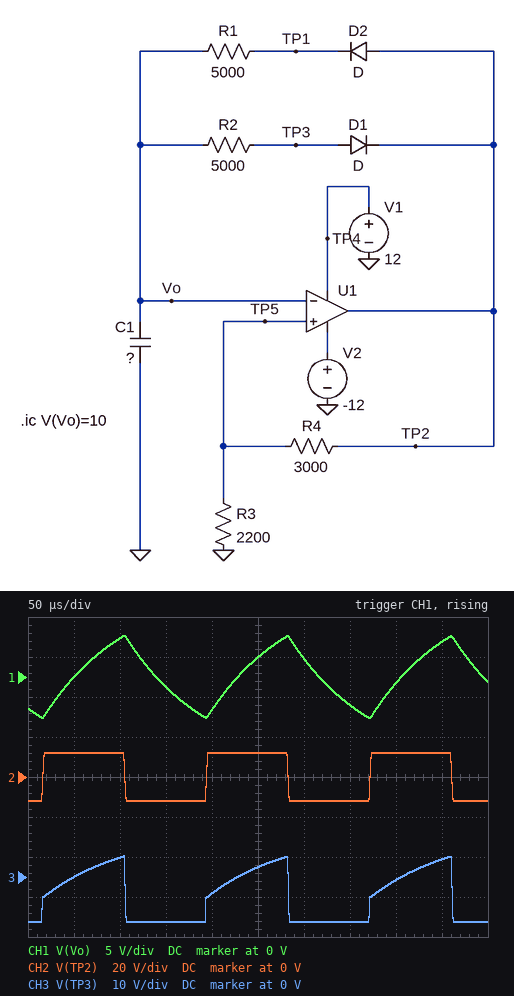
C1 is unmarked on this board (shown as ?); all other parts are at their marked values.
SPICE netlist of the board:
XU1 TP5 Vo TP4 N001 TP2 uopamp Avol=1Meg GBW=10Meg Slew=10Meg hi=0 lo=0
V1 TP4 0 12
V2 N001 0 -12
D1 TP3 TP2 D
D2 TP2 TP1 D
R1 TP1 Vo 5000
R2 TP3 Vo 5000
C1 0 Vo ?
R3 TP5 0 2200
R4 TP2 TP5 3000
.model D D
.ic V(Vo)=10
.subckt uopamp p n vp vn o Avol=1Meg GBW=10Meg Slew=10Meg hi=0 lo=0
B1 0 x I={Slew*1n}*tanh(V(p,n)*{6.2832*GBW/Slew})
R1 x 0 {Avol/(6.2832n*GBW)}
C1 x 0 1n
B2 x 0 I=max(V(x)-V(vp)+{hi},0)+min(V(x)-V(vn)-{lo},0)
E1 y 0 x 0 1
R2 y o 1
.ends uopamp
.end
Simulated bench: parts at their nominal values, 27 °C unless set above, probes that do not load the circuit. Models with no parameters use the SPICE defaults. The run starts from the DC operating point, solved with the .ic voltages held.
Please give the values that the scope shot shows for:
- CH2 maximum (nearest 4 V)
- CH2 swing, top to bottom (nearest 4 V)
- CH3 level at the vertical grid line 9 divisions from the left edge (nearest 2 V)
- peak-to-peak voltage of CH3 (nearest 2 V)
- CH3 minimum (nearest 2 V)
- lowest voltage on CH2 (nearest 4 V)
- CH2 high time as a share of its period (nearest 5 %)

12 V
24 V
4 V
16 V
-12 V
-12 V
50 %
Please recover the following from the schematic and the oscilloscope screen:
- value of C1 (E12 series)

18 nF
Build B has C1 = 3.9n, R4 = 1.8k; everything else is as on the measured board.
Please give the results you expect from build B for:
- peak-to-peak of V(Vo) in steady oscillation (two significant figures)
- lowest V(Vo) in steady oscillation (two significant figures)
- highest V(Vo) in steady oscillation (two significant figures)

13 V
-6.7 V
6.7 V
